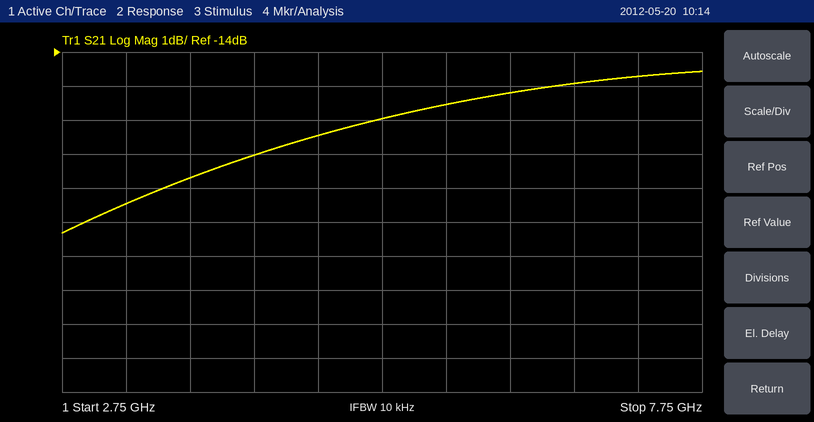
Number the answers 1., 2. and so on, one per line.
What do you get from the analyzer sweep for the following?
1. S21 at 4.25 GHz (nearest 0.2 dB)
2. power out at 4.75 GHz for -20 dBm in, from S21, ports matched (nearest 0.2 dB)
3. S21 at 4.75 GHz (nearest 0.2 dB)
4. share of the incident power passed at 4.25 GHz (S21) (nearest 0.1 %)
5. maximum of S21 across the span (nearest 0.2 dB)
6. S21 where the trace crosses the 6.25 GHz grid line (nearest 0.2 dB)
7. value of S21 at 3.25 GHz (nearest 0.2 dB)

1. -17.0 dB
2. -36.4 dBm
3. -16.4 dB
4. 2.0 %
5. -14.6 dB
6. -15.2 dB
7. -18.4 dB
